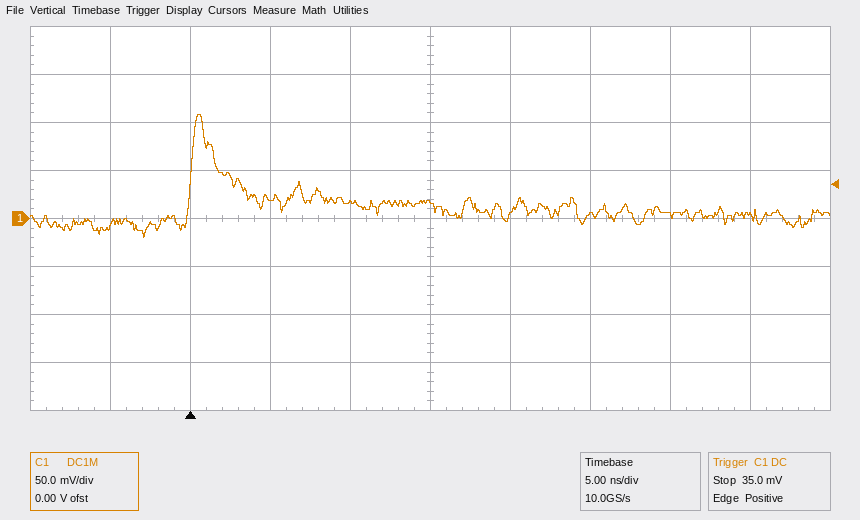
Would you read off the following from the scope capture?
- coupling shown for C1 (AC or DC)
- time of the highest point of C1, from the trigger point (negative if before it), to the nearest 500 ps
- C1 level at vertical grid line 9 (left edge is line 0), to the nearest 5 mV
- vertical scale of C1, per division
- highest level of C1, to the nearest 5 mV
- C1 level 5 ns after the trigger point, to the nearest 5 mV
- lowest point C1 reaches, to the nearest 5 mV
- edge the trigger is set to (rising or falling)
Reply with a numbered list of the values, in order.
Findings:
1. DC
2. +500 ps
3. 0 mV
4. 50 mV
5. 110 mV
6. 20 mV
7. -20 mV
8. rising
